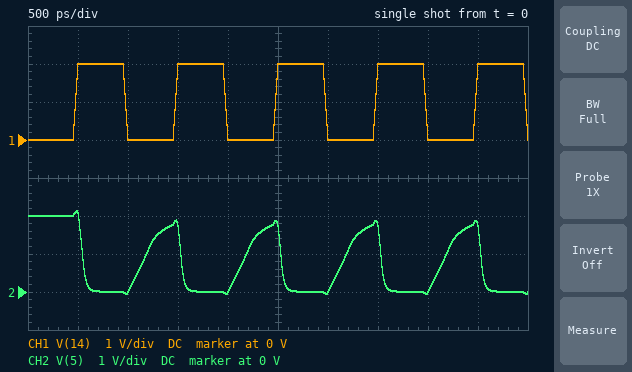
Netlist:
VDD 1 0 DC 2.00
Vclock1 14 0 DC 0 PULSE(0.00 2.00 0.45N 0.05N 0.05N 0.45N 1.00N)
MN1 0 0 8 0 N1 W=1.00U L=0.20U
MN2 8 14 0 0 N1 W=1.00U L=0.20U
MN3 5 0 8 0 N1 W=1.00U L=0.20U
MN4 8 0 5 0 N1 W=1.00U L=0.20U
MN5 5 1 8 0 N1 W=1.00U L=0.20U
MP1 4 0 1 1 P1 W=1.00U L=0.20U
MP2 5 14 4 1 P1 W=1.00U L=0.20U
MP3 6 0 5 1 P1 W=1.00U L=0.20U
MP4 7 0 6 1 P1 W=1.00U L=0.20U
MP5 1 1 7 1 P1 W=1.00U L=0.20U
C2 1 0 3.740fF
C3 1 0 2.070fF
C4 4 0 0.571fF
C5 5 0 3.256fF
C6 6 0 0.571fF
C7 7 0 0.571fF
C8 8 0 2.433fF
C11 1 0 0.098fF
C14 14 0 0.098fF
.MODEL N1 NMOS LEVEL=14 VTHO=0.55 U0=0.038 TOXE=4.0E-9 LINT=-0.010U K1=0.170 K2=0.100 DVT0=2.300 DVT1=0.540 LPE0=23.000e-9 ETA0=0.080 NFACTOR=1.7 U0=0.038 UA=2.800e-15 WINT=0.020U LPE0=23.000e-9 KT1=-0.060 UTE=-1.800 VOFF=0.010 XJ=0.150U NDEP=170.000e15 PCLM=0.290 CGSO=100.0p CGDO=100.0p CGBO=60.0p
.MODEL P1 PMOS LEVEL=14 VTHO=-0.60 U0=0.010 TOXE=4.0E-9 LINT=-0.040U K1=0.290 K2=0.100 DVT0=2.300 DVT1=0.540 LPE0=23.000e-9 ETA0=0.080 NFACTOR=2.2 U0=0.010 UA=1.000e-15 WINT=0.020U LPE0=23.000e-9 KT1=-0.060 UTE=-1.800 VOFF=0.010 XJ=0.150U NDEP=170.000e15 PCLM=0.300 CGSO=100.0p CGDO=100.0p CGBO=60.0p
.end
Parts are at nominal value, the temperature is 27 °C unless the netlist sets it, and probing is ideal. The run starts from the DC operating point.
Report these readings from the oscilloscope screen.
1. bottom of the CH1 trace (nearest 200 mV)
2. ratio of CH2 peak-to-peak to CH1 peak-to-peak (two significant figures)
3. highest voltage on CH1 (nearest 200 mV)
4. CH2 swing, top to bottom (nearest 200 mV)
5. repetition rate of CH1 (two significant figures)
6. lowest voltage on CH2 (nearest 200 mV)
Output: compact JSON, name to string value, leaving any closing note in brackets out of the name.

{"bottom of the CH1 trace": "0 V", "ratio of CH2 peak-to-peak to CH1 peak-to-peak": "1.1", "highest voltage on CH1": "2.0 V", "CH2 swing, top to bottom": "2.2 V", "repetition rate of CH1": "1.0 GHz", "lowest voltage on CH2": "0 V"}
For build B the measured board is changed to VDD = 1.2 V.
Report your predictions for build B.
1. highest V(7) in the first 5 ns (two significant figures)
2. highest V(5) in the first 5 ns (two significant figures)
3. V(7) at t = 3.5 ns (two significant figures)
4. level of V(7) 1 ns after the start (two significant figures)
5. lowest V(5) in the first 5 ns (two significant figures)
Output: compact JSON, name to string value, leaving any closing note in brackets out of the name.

{"highest V(7) in the first 5 ns": "1.2 V", "highest V(5) in the first 5 ns": "1.3 V", "V(7) at t = 3.5 ns": "860 mV", "level of V(7) 1 ns after the start": "940 mV", "lowest V(5) in the first 5 ns": "-76 mV"}
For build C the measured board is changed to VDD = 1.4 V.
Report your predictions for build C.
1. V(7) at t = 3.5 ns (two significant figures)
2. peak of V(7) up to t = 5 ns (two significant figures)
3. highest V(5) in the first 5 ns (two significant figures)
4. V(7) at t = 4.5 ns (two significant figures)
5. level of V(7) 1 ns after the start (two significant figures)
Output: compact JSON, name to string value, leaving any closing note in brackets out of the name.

{"V(7) at t = 3.5 ns": "890 mV", "peak of V(7) up to t = 5 ns": "1.4 V", "highest V(5) in the first 5 ns": "1.5 V", "V(7) at t = 4.5 ns": "880 mV", "level of V(7) 1 ns after the start": "980 mV"}
